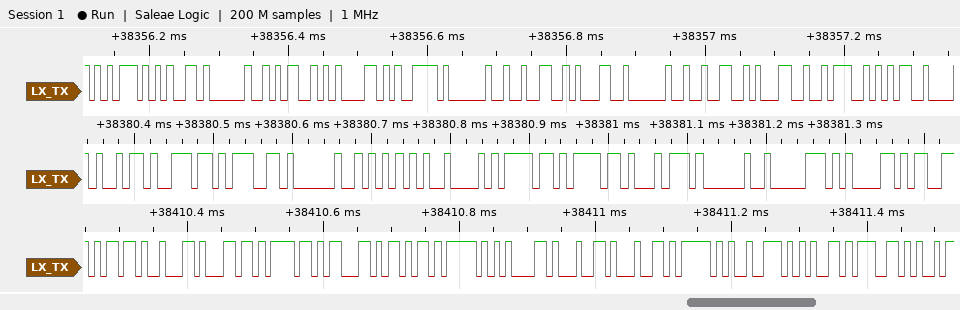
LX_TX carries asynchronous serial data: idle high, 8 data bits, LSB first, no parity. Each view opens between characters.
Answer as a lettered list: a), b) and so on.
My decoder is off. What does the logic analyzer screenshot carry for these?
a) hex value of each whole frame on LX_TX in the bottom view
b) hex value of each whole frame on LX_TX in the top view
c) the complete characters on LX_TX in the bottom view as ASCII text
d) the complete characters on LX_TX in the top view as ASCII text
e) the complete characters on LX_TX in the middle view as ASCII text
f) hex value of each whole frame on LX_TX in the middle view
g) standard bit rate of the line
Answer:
a) 6D, 62, 6C, 6F, 63, 6B, 5F, 61, 64, 64, 5F, 72, 65, 67
b) 75, 65, 20, 4D, 61, 79, 20, 32, 31, 20, 32, 31, 3A, 35
c) "mblock_add_reg"
d) "ue May 21 21:5"
e) "ing UBoot pa"
f) 69, 6E, 67, 20, 55, 42, 6F, 6F, 74, 20, 70, 61
g) 115200 baud
